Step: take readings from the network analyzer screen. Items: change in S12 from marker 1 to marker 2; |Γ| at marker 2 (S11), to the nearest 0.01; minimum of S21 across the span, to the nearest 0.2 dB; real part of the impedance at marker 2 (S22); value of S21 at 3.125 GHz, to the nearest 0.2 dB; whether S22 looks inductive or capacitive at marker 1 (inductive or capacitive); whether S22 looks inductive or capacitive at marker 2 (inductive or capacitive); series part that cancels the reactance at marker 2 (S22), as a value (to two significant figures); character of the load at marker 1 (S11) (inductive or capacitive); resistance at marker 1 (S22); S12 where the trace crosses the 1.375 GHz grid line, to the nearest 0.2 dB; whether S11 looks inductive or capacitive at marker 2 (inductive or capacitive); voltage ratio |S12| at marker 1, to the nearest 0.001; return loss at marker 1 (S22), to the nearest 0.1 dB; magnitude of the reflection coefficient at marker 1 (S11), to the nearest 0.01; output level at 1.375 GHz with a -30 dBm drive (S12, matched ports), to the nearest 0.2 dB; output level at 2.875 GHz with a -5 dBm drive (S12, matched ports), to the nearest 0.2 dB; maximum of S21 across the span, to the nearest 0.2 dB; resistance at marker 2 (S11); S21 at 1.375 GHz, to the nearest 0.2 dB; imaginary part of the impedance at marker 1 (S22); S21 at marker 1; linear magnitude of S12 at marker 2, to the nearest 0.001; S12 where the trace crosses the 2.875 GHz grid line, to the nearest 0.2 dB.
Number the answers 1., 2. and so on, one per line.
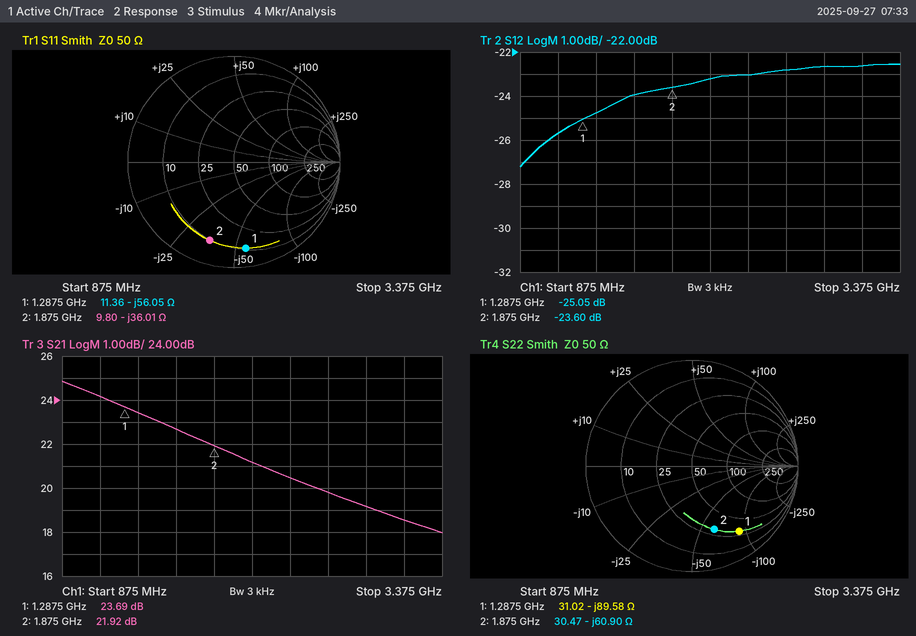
1. 1.45 dB
2. 0.77
3. 18.0 dB
4. 30.47 Ω
5. 18.6 dB
6. capacitive
7. capacitive
8. 5.2 nH
9. capacitive
10. 31.02 Ω
11. -24.8 dB
12. capacitive
13. 0.056
14. 2.4 dB
15. 0.82
16. -54.8 dBm
17. -27.6 dBm
18. 24.8 dB
19. 9.80 Ω
20. 23.4 dB
21. -89.58 Ω
22. 23.69 dB
23. 0.066
24. -22.6 dB
